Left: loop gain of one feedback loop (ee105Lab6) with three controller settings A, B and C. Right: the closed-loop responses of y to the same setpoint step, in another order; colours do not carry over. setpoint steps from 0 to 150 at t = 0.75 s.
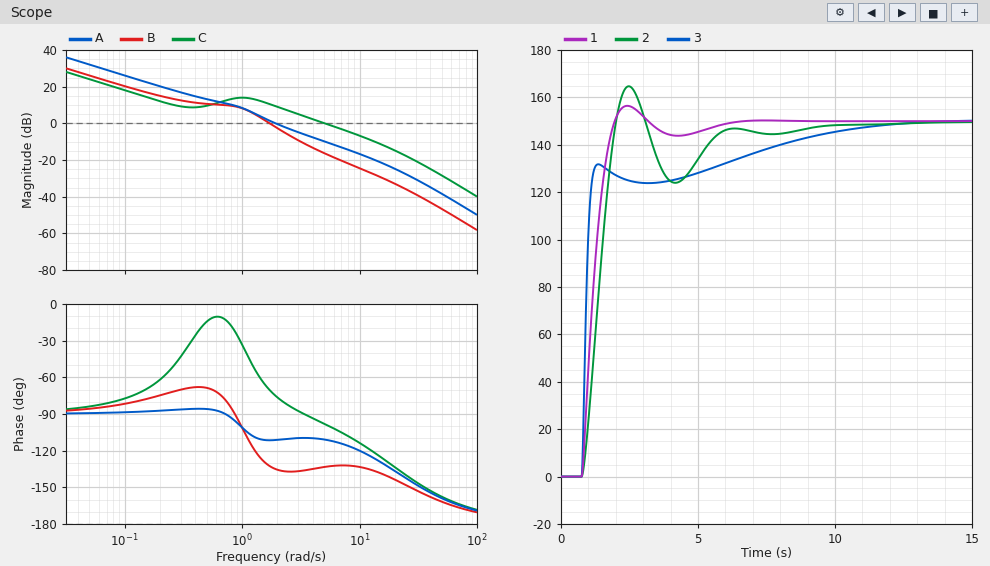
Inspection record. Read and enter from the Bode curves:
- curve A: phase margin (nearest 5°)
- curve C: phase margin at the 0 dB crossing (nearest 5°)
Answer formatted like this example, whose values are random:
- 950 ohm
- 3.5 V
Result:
- 70°
- 80°
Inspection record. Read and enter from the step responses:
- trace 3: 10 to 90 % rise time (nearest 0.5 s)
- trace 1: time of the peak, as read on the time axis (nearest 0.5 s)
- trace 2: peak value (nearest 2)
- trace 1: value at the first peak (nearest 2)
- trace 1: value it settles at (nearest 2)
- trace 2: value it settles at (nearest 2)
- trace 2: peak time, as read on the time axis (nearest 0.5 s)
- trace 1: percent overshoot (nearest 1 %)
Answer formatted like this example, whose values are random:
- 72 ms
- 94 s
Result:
- 6.0 s
- 2.5 s
- 164
- 156
- 150
- 150
- 2.5 s
- 4 %
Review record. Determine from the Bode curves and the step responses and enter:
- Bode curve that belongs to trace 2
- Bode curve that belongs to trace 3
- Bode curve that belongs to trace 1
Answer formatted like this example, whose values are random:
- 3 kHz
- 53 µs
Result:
- B
- C
- A
